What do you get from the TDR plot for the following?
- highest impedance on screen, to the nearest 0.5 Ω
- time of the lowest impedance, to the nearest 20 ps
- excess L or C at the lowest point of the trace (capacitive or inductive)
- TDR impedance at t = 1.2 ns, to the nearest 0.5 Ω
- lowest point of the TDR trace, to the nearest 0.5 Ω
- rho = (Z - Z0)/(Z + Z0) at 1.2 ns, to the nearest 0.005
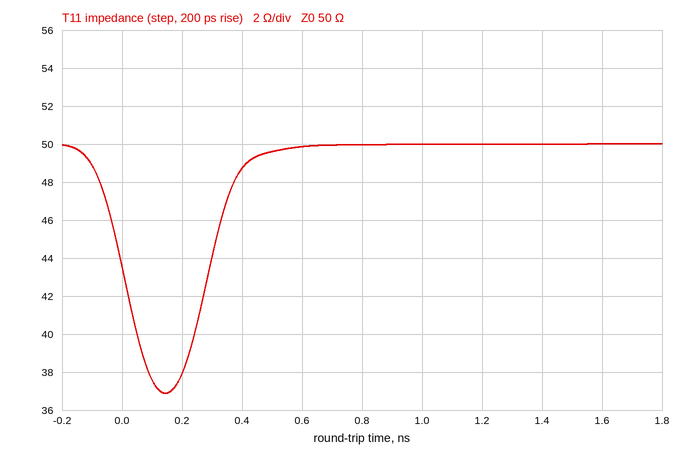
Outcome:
50.0 Ω
140 ps
capacitive
50.0 Ω
37.0 Ω
0.000
